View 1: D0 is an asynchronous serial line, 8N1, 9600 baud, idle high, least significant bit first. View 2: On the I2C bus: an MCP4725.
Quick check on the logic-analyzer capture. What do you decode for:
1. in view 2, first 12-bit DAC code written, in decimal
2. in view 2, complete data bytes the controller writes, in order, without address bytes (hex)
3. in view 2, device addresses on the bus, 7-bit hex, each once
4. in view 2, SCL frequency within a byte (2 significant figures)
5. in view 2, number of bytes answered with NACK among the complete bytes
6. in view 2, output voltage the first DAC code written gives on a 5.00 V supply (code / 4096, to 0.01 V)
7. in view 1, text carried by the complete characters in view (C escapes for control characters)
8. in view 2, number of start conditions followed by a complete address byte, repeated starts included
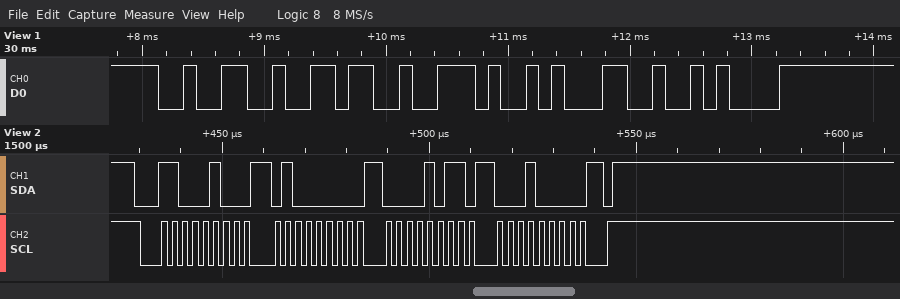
177
40 0B 10
0x62
400 kHz
0
0.22 V
"26.1\n"
1
